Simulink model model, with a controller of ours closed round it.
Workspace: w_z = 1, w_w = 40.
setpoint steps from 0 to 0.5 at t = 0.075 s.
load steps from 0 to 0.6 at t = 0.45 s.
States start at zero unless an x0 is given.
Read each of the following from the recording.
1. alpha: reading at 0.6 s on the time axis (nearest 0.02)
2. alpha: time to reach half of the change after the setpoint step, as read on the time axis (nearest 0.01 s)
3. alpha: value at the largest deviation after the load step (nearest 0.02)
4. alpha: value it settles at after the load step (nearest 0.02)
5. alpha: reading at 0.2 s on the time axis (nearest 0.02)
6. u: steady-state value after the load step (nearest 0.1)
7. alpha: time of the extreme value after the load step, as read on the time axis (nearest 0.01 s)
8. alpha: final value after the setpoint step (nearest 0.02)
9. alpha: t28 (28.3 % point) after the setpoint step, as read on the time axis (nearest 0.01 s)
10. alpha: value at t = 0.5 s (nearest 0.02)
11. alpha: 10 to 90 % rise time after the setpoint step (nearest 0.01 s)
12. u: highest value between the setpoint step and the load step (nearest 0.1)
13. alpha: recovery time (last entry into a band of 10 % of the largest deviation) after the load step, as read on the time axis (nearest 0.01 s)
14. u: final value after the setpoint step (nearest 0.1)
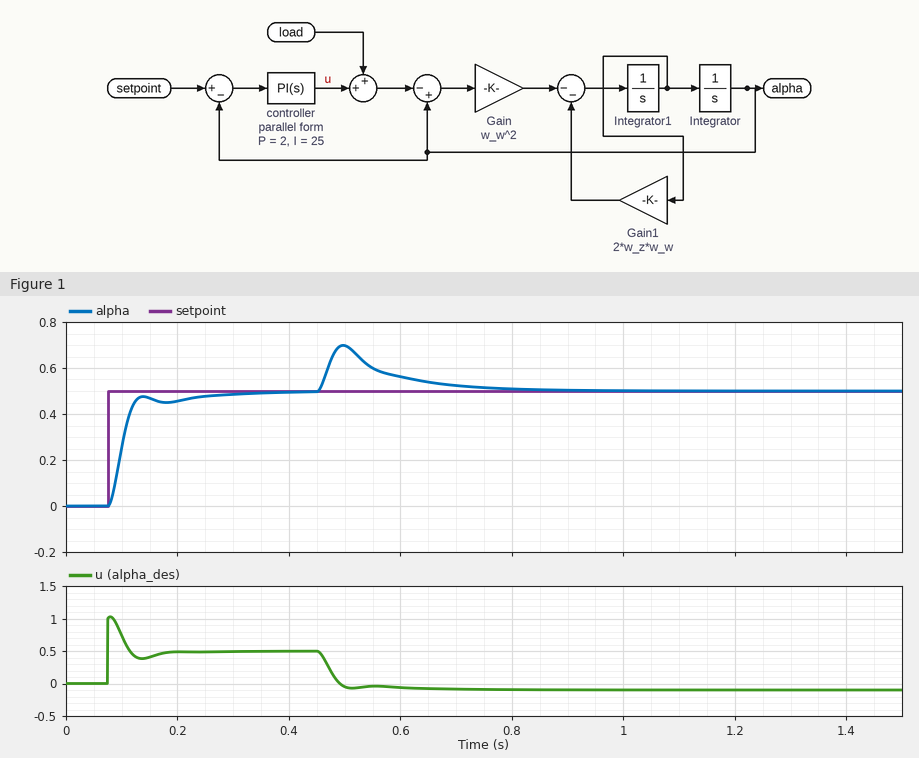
0.56
0.10 s
0.70
0.50
0.46
-0.1
0.50 s
0.50
0.09 s
0.70
0.04 s
1.0
0.72 s
0.5
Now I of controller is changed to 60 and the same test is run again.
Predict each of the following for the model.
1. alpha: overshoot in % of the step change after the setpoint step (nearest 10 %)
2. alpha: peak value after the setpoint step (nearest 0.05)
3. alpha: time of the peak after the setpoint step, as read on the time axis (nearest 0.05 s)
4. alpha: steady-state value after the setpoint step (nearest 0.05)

20 %
0.60
0.15 s
0.50
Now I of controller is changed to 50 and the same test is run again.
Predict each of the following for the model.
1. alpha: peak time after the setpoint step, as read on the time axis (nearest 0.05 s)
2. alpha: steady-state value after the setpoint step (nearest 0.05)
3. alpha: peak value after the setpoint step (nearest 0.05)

0.15 s
0.50
0.55
